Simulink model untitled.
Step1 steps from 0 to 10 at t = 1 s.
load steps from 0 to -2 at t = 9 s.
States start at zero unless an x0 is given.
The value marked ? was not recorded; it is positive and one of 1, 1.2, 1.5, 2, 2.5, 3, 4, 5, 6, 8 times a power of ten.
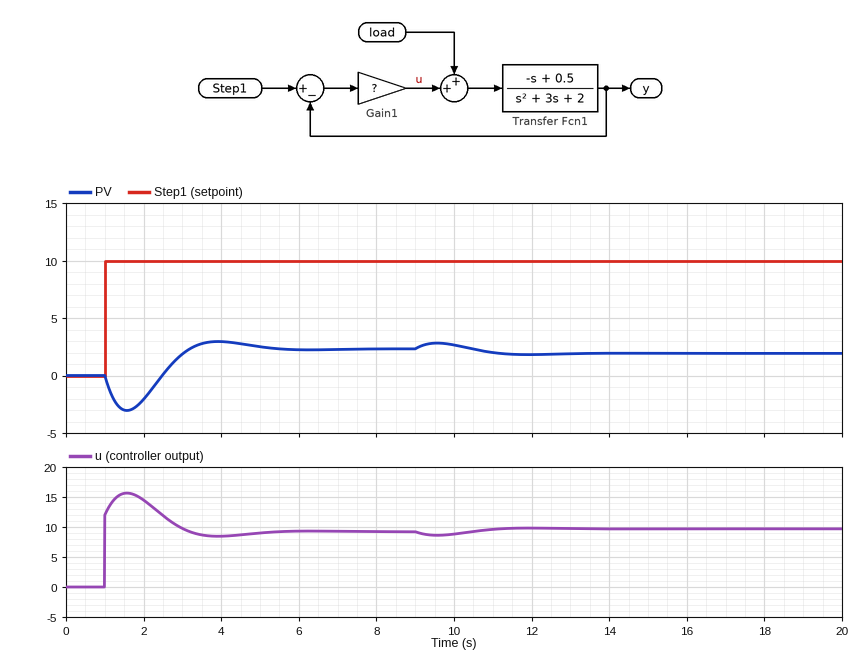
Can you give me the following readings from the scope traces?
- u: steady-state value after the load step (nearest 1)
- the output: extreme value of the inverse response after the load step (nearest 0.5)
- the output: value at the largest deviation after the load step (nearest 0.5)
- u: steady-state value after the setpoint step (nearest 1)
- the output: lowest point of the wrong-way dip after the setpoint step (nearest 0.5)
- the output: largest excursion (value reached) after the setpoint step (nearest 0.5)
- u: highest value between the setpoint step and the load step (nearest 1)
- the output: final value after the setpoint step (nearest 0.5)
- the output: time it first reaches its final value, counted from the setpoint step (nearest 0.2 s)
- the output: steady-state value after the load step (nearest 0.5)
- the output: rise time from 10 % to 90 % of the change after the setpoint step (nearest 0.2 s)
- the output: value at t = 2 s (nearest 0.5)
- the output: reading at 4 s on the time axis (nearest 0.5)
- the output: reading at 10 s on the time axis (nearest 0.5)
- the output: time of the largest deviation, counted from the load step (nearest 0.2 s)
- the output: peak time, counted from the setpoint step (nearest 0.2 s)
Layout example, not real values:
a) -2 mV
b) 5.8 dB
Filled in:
a) 10
b) 3.0
c) 2.0
d) 9
e) -3.0
f) 3.0
g) 16
h) 2.5
i) 2.2 s
j) 2.0
k) 0.6 s
l) -2.0
m) 3.0
n) 2.5
o) 3.0 s
p) 3.0 s
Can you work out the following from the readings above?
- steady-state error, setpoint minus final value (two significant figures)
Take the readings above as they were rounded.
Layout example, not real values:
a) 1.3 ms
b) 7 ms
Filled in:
a) 7.5
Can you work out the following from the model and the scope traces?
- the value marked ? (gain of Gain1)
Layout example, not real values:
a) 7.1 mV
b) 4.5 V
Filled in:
a) 1.2
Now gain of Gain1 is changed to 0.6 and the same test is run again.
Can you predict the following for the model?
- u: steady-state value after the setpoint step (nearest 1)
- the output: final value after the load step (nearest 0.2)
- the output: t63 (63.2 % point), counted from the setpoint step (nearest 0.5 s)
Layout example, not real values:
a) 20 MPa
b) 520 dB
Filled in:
a) 5
b) 0.8
c) 2.0 s
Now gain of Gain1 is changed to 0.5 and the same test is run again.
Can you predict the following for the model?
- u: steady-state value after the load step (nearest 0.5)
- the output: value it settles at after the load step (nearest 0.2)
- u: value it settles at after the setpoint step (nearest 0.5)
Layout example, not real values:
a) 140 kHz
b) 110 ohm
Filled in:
a) 4.5
b) 0.6
c) 4.5
